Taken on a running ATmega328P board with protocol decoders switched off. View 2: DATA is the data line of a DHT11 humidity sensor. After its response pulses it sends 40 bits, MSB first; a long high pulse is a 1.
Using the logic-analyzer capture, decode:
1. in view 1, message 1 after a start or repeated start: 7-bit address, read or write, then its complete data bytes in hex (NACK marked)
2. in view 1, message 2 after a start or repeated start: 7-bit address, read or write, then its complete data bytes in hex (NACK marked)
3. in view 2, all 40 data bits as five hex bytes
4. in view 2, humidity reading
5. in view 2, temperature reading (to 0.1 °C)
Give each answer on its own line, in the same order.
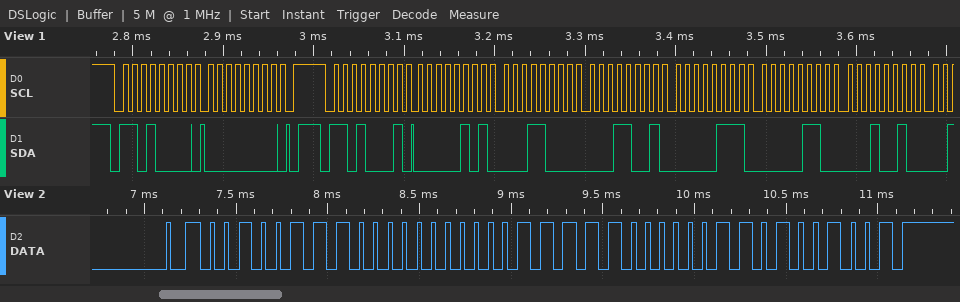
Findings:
0x68 write: 00
0x68 read: 05 18 19 07 06 12
27 00 1F 03 49
39 %
31.3 °C
